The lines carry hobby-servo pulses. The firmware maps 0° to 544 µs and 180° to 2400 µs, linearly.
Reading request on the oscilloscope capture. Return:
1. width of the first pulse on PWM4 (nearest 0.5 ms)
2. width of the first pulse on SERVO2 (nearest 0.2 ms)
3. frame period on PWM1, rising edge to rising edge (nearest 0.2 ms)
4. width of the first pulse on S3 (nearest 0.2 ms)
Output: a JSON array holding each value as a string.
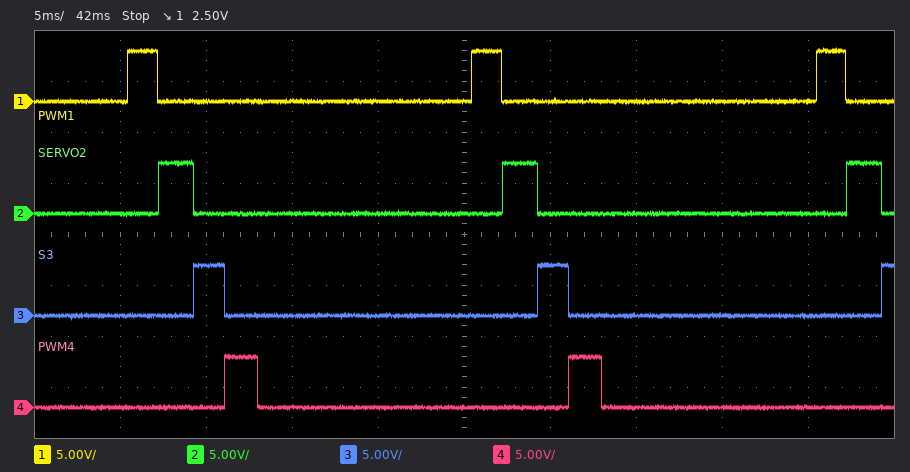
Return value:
["2.0 ms", "2.0 ms", "20.0 ms", "1.8 ms"]
